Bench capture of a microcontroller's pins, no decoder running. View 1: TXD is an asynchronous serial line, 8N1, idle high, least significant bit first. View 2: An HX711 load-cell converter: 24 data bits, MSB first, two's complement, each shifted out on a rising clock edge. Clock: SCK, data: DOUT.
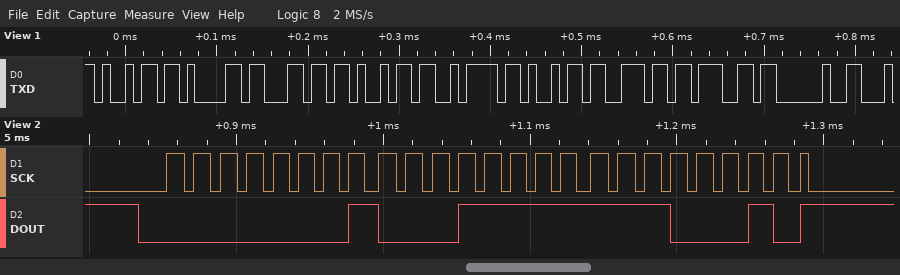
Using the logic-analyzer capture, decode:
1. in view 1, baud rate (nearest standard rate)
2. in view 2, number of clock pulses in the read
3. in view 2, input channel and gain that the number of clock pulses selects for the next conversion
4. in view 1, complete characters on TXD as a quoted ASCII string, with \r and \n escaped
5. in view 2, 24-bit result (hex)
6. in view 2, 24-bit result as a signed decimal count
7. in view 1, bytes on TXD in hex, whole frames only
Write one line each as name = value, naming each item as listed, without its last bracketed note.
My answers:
in view 1, baud rate = 115200 baud
in view 2, number of clock pulses in the read = 25
in view 2, input channel and gain that the number of clock pulses selects for the next conversion = channel A, gain 128
in view 1, complete characters on TXD as a quoted ASCII string, with \r and \n escaped = "ializing "
in view 2, 24-bit result = 0x011FE2
in view 2, 24-bit result as a signed decimal count = 73698
in view 1, bytes on TXD in hex, whole frames only = 0x69 0x61 0x6C 0x69 0x7A 0x69 0x6E 0x67 0x20
